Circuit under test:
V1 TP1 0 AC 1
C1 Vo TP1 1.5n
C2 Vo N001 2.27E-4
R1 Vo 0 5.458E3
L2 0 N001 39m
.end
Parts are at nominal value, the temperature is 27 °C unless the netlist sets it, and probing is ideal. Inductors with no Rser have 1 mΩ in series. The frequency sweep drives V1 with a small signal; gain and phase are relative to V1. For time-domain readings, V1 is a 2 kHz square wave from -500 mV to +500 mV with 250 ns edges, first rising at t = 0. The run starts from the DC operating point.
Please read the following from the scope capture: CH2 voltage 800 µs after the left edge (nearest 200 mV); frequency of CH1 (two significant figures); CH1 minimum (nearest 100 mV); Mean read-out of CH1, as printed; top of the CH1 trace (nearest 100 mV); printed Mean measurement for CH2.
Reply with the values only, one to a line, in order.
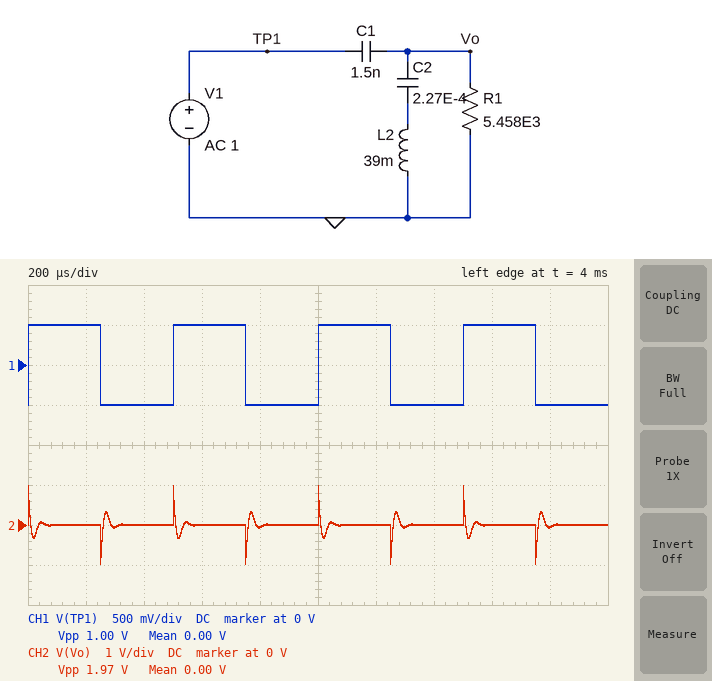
0 V
2.0 kHz
-500 mV
0.00 V
500 mV
0.00 V
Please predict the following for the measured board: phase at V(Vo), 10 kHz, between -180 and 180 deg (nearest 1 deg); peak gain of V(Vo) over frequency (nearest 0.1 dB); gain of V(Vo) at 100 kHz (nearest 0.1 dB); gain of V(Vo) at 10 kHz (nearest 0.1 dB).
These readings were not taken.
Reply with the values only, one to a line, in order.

150 deg
1.7 dB
0.2 dB
-11.7 dB
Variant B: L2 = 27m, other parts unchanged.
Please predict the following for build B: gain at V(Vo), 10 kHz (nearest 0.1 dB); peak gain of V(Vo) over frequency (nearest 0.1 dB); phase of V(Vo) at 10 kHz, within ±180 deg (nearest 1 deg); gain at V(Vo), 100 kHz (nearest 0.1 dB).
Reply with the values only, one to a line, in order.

-15.0 dB
2.9 dB
160 deg
0.4 dB
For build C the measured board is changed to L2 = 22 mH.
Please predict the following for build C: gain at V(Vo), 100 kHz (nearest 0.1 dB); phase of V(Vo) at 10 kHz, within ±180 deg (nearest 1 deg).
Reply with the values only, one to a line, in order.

0.5 dB
164 deg
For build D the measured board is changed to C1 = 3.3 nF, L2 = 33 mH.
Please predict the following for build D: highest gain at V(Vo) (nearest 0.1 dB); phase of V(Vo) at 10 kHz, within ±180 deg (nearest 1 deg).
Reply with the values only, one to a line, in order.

5.1 dB
146 deg
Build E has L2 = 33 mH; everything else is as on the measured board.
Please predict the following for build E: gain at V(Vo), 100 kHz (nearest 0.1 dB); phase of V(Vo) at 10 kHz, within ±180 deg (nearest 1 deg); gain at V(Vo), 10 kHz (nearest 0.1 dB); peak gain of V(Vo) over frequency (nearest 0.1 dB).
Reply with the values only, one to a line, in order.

0.3 dB
155 deg
-13.2 dB
2.2 dB
